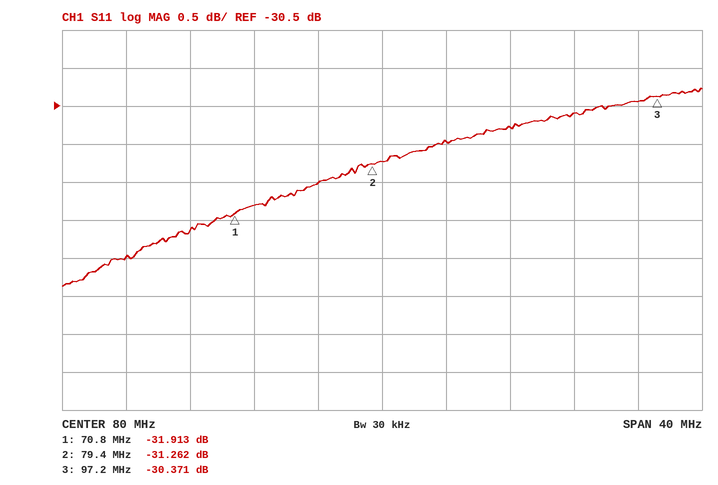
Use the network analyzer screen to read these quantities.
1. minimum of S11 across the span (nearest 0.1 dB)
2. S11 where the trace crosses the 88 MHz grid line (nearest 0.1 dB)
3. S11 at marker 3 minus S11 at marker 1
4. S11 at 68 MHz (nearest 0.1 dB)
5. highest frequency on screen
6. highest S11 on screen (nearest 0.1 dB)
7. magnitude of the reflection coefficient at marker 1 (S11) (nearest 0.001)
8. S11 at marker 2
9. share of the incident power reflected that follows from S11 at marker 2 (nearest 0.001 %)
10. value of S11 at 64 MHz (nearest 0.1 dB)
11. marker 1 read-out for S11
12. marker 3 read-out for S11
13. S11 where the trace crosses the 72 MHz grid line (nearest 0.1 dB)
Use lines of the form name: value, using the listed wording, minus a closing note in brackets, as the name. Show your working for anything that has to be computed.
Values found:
minimum of S11 across the span: -32.9 dB
S11 where the trace crosses the 88 MHz grid line: -30.8 dB
S11 at marker 3 minus S11 at marker 1: -30.371 − (-31.913) = 1.542 dB
S11 at 68 MHz: -32.1 dB
highest frequency on screen: 100 MHz
highest S11 on screen: -30.3 dB
magnitude of the reflection coefficient at marker 1 (S11): 10^(-31.913/20) ≈ 0.025
S11 at marker 2: -31.262 dB
share of the incident power reflected that follows from S11 at marker 2: 10^(-31.262/10) ≈ 0.075 %
value of S11 at 64 MHz: -32.5 dB
marker 1 read-out for S11: -31.913 dB
marker 3 read-out for S11: -30.371 dB
S11 where the trace crosses the 72 MHz grid line: -31.8 dB
